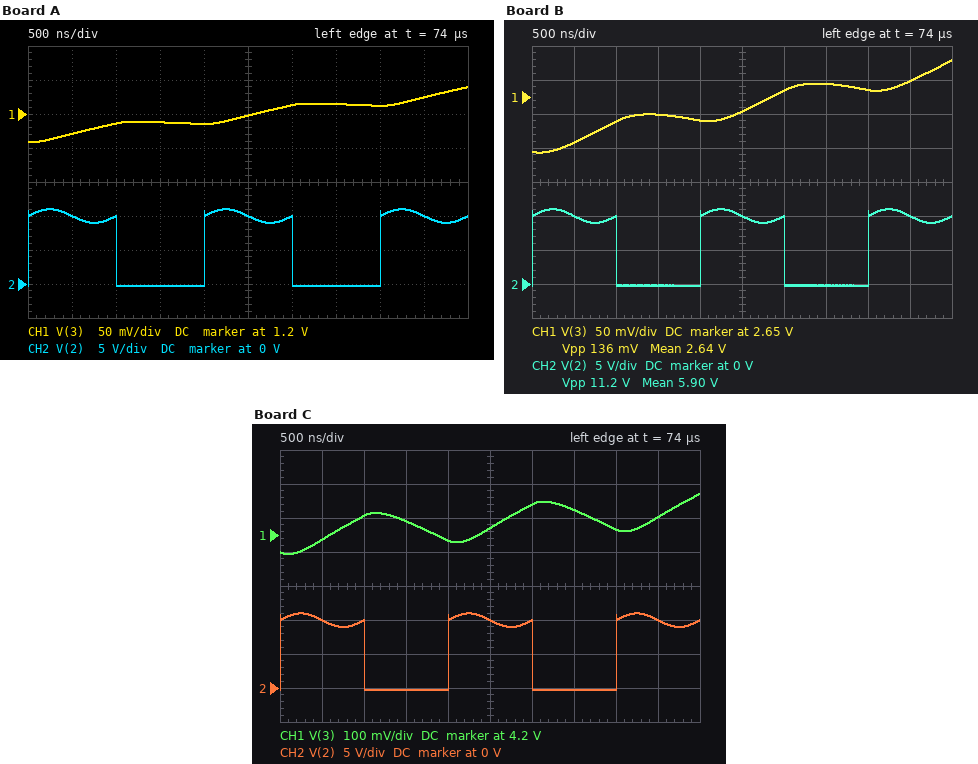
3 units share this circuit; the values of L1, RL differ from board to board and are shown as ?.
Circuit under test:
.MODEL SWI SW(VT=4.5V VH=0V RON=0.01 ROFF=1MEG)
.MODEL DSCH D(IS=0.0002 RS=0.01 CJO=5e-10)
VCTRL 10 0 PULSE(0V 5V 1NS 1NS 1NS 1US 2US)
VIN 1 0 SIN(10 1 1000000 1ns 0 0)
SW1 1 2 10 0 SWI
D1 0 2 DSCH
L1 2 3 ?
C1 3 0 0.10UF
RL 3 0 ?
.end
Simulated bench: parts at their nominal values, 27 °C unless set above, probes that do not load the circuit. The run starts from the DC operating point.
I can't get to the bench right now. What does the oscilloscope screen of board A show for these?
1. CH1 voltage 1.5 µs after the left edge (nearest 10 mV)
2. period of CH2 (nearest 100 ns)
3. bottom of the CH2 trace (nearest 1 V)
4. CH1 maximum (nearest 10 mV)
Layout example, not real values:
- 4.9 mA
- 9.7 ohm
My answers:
- 1.19 V
- 2.0 µs
- 0 V
- 1.24 V
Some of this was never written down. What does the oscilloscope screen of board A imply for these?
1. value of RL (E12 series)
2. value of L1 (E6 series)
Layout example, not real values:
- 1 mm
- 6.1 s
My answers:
- 1.2 Ω
- 330 µH
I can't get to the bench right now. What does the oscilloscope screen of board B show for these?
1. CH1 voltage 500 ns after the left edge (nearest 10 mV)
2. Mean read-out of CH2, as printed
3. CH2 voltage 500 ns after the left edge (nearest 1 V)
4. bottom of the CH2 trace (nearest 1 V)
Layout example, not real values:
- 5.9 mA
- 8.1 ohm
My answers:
- 2.58 V
- 5.90 V
- 10 V
- 0 V
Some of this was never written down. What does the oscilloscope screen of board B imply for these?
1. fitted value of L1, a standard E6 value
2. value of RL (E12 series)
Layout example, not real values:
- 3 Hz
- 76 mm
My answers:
- 330 µH
- 3.3 Ω
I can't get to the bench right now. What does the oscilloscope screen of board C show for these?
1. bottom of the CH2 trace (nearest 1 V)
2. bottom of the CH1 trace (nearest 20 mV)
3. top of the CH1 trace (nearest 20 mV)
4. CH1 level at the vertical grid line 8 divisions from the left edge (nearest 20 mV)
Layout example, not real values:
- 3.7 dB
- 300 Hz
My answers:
- 0 V
- 4.14 V
- 4.32 V
- 4.22 V
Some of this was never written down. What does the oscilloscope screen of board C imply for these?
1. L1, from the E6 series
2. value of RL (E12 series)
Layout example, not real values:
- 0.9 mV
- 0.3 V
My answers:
- 68 µH
- 1.8 Ω
